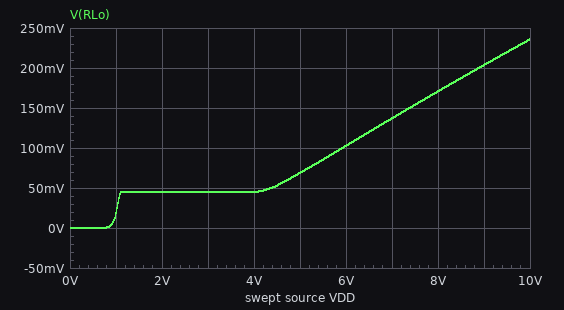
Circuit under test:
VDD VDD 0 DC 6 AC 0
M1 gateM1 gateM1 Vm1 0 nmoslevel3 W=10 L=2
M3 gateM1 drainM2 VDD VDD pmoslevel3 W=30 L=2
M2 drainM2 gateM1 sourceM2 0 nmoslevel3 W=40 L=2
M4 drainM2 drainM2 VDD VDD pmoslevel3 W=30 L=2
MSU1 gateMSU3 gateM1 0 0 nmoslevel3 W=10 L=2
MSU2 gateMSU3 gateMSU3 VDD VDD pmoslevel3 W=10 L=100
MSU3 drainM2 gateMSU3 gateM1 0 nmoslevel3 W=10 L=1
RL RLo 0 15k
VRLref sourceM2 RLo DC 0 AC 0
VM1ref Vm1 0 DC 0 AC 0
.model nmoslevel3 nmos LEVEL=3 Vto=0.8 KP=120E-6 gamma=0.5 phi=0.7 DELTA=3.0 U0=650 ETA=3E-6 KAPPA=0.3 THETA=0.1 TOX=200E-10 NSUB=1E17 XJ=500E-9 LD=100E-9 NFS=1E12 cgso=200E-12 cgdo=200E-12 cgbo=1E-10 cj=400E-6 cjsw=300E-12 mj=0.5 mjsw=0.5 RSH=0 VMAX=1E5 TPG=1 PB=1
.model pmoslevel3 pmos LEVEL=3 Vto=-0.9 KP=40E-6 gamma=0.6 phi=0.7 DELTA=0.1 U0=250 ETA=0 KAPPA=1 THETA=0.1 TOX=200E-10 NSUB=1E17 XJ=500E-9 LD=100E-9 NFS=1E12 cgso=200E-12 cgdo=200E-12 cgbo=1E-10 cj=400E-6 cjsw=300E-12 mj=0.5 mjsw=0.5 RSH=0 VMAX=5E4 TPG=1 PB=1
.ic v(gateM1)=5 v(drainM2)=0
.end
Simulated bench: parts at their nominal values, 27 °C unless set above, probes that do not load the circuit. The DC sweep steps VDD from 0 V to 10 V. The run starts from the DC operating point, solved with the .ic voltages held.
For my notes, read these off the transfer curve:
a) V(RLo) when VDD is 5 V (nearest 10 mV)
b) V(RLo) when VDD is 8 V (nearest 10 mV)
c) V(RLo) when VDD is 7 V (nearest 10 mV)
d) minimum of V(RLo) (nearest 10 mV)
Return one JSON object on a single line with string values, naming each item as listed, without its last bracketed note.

{"V(RLo) when VDD is 5 V": "70 mV", "V(RLo) when VDD is 8 V": "170 mV", "V(RLo) when VDD is 7 V": "140 mV", "minimum of V(RLo)": "0 V"}
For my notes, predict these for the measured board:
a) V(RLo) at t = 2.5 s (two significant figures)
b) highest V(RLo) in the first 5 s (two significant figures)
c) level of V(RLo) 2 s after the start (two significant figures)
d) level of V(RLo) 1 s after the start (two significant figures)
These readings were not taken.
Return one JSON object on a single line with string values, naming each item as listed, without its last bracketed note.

{"V(RLo) at t = 2.5 s": "19 mV", "highest V(RLo) in the first 5 s": "44 mV", "level of V(RLo) 2 s after the start": "14 mV", "level of V(RLo) 1 s after the start": "6.4 mV"}
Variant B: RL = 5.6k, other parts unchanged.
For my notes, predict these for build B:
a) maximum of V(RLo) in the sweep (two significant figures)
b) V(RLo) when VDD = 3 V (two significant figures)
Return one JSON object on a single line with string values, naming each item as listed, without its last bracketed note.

{"maximum of V(RLo) in the sweep": "190 mV", "V(RLo) when VDD = 3 V": "110 mV"}
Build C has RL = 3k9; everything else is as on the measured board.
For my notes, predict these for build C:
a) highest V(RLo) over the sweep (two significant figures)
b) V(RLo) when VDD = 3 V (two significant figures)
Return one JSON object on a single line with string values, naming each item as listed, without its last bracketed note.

{"highest V(RLo) over the sweep": "170 mV", "V(RLo) when VDD = 3 V": "160 mV"}
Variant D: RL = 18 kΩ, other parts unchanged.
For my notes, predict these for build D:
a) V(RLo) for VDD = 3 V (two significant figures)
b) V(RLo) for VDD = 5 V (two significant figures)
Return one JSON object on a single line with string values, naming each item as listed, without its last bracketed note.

{"V(RLo) for VDD = 3 V": "46 mV", "V(RLo) for VDD = 5 V": "72 mV"}
